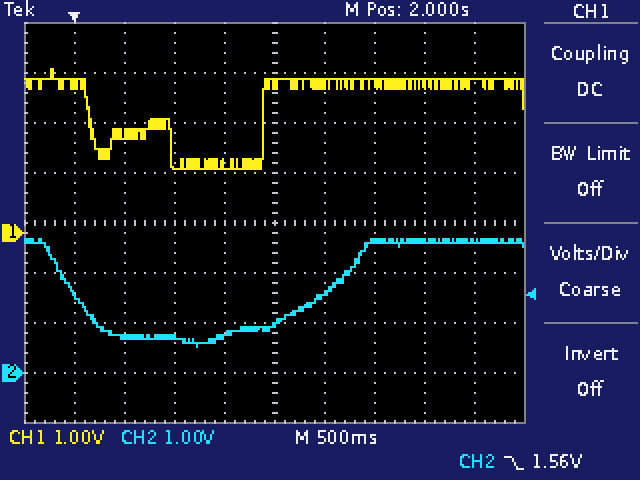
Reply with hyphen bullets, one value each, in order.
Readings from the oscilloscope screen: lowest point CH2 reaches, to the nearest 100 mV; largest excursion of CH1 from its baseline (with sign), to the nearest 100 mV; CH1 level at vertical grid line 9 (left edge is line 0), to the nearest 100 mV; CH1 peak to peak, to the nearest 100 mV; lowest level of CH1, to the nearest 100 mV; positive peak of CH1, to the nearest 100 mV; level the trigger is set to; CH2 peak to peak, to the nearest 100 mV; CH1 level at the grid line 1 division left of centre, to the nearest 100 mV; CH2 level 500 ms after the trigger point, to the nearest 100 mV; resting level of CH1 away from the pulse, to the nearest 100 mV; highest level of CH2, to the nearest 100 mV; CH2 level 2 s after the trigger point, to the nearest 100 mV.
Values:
- 500 mV
- -1.7 V
- 3.1 V
- 2.0 V
- 1.3 V
- 3.3 V
- 1.56 V
- 2.2 V
- 1.4 V
- 700 mV
- 3.0 V
- 2.7 V
- 1.0 V
